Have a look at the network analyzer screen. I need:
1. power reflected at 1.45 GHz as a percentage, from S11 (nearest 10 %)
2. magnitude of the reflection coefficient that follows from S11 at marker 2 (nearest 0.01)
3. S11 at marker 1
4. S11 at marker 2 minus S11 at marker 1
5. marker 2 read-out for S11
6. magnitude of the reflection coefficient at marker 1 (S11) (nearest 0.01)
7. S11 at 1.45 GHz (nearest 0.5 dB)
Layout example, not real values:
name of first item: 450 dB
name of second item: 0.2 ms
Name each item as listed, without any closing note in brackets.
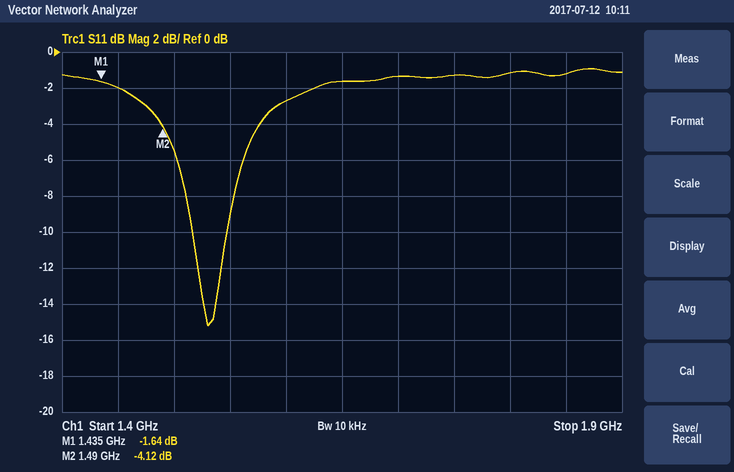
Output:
power reflected at 1.45 GHz as a percentage, from S11: 60 %
magnitude of the reflection coefficient that follows from S11 at marker 2: 0.62
S11 at marker 1: -1.64 dB
S11 at marker 2 minus S11 at marker 1: -2.48 dB
marker 2 read-out for S11: -4.12 dB
magnitude of the reflection coefficient at marker 1 (S11): 0.83
S11 at 1.45 GHz: -2.0 dB
